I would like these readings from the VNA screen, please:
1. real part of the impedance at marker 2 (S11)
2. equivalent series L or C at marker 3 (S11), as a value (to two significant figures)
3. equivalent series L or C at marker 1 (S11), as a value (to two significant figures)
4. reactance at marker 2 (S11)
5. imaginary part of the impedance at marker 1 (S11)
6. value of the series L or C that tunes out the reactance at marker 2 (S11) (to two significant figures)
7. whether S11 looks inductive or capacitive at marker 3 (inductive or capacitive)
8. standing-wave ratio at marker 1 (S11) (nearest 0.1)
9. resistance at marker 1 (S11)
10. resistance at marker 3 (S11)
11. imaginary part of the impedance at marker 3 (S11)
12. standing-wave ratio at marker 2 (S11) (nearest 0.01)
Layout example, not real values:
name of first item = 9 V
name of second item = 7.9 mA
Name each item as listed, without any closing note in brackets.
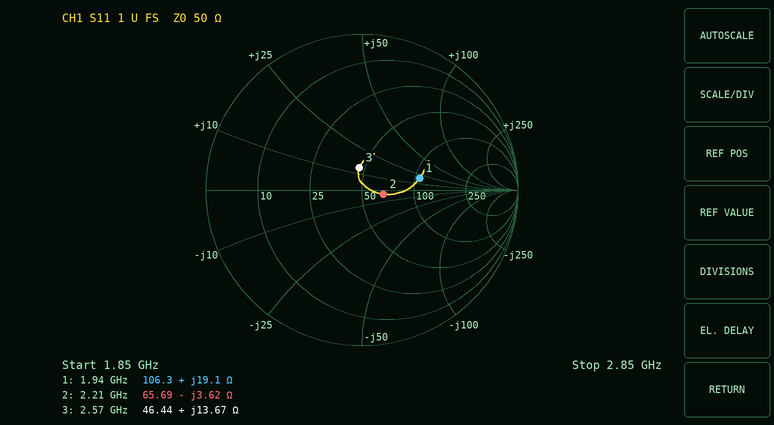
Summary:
real part of the impedance at marker 2 = 65.69 Ω
equivalent series L or C at marker 3 (S11), as a value = 850 pH
equivalent series L or C at marker 1 (S11), as a value = 1.6 nH
reactance at marker 2 = -3.62 Ω
imaginary part of the impedance at marker 1 = +19.1 Ω
value of the series L or C that tunes out the reactance at marker 2 (S11) = 260 pH
whether S11 looks inductive or capacitive at marker 3 = inductive
standing-wave ratio at marker 1 (S11) = 2.2
resistance at marker 1 = 106.3 Ω
resistance at marker 3 = 46.44 Ω
imaginary part of the impedance at marker 3 = +13.67 Ω
standing-wave ratio at marker 2 (S11) = 1.32
